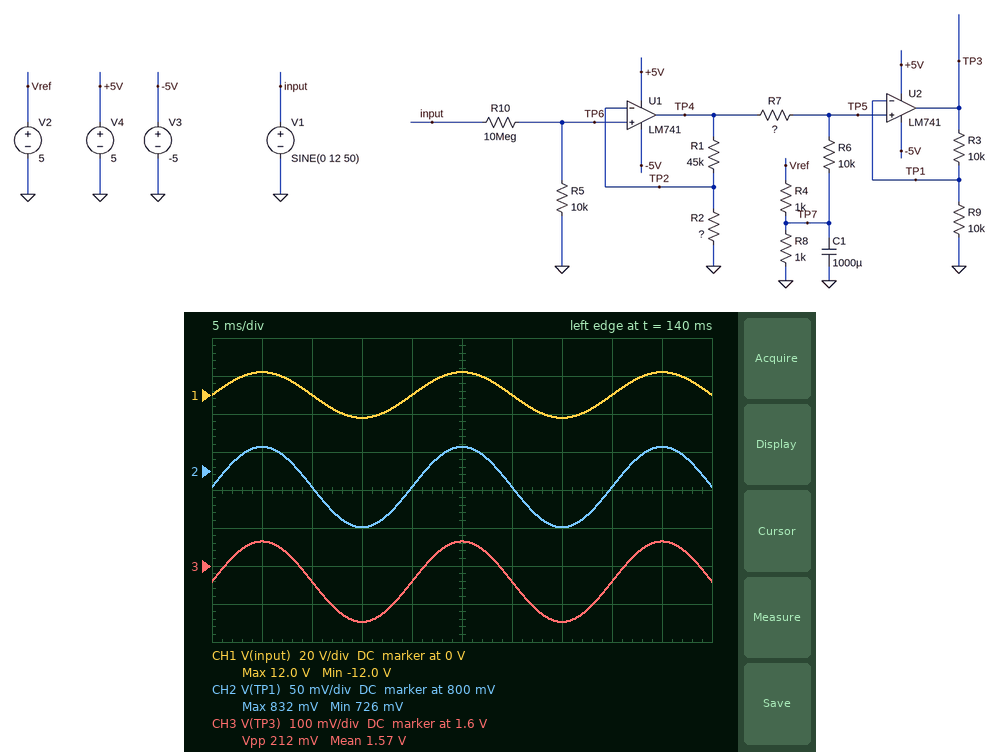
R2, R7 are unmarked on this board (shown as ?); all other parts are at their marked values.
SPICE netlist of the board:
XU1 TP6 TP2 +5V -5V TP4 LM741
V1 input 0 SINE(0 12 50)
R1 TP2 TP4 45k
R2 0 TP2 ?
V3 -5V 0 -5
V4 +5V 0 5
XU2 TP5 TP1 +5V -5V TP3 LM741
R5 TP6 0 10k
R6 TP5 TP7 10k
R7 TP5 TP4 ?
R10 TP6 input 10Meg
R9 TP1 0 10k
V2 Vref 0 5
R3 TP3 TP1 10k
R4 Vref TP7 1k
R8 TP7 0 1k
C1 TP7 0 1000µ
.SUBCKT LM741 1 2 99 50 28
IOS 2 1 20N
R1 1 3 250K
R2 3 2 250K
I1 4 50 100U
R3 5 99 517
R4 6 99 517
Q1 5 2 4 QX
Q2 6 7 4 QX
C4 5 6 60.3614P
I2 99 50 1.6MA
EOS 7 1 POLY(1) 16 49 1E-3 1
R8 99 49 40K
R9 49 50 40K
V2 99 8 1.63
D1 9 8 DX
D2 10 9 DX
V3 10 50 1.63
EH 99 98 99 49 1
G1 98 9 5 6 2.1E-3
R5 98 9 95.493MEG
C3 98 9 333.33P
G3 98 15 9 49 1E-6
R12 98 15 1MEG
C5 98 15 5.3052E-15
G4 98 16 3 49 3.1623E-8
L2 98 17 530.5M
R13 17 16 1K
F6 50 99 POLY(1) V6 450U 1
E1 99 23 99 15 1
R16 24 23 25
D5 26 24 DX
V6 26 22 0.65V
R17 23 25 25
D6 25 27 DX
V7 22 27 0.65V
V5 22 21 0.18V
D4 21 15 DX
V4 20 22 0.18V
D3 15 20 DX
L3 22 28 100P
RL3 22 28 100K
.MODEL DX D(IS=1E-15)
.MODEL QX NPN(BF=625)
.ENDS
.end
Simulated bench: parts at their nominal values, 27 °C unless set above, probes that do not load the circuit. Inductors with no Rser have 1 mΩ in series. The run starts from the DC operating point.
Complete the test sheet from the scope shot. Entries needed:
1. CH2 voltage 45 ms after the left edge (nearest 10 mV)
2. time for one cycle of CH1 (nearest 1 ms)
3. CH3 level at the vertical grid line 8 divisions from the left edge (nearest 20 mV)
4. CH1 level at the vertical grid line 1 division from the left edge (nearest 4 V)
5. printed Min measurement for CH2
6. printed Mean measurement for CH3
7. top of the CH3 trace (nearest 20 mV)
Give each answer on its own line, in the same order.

830 mV
20 ms
1.56 V
12 V
726 mV
1.57 V
1.66 V
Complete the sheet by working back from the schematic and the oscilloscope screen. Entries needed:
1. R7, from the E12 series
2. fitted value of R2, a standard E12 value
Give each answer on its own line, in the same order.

4.7 kΩ
8.2 kΩ
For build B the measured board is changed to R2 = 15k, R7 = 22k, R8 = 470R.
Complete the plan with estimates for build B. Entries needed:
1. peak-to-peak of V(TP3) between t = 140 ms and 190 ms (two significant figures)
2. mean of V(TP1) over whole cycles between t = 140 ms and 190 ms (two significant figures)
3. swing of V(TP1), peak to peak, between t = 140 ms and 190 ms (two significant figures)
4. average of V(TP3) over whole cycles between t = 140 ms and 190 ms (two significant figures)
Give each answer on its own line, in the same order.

60 mV
1.1 V
30 mV
2.2 V
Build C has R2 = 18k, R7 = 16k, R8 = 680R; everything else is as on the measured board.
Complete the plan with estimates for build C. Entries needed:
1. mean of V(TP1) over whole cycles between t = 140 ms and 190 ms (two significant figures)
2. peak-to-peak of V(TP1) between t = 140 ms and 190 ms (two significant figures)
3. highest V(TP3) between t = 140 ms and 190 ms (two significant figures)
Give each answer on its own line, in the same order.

1.2 V
32 mV
2.5 V
